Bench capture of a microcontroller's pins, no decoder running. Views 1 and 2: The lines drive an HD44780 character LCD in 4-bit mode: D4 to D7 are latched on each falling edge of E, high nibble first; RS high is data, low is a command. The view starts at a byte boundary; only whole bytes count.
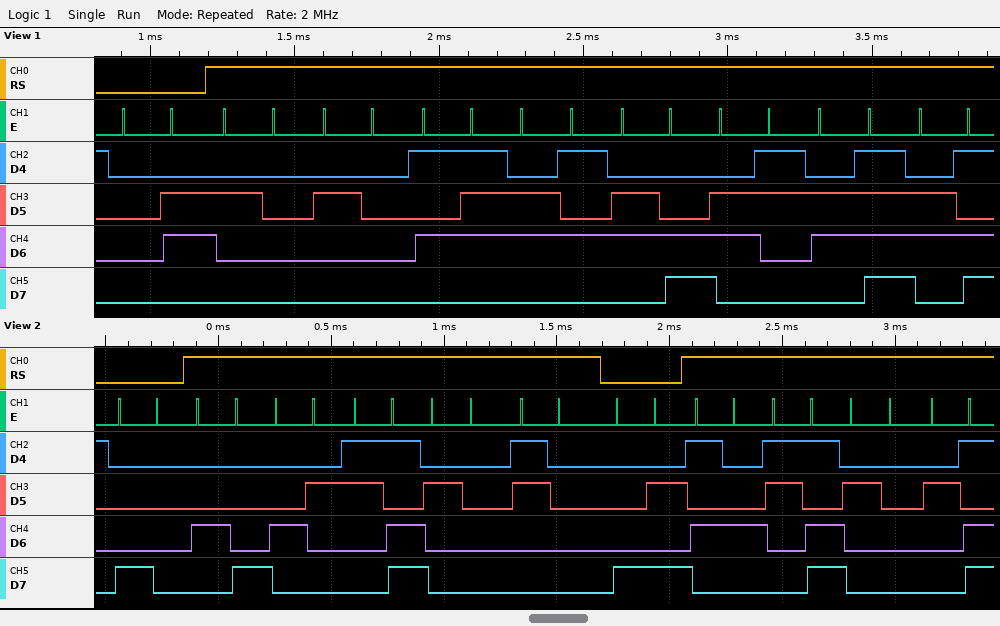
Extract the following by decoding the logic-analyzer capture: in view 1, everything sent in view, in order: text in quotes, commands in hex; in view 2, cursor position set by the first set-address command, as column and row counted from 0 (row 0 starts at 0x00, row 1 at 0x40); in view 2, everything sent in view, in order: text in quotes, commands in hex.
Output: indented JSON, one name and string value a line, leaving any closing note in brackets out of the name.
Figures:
{
  "in view 1, everything sent in view, in order: text in quotes, commands in hex": "0x06 \"  Welcom\"",
  "in view 2, cursor position set by the first set-address command, as column and row counted from 0": "column 0, row 0",
  "in view 2, everything sent in view, in order: text in quotes, commands in hex": "0x80 \"HB= 0\" 0x8A \"T= -\""
}
